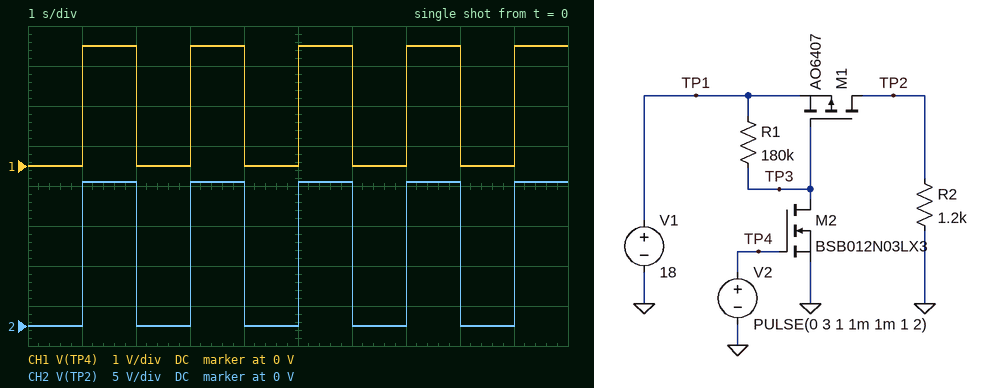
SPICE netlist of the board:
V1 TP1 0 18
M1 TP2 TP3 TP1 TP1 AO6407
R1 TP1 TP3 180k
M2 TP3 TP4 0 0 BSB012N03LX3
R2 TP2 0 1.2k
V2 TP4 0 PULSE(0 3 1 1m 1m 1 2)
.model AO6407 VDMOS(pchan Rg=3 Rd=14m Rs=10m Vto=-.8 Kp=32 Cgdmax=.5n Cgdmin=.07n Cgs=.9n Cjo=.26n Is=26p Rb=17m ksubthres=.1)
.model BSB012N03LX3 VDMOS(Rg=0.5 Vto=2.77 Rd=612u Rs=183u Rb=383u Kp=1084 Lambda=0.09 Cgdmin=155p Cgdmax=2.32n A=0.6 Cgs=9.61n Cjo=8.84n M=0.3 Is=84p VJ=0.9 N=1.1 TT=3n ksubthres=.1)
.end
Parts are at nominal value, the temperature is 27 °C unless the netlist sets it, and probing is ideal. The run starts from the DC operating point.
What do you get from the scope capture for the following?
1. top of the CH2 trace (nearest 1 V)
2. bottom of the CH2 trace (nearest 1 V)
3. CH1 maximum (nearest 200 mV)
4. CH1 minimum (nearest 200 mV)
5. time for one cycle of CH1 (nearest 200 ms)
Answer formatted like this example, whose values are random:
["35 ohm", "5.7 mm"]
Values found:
["18 V", "0 V", "3.0 V", "0 V", "2.0 s"]
